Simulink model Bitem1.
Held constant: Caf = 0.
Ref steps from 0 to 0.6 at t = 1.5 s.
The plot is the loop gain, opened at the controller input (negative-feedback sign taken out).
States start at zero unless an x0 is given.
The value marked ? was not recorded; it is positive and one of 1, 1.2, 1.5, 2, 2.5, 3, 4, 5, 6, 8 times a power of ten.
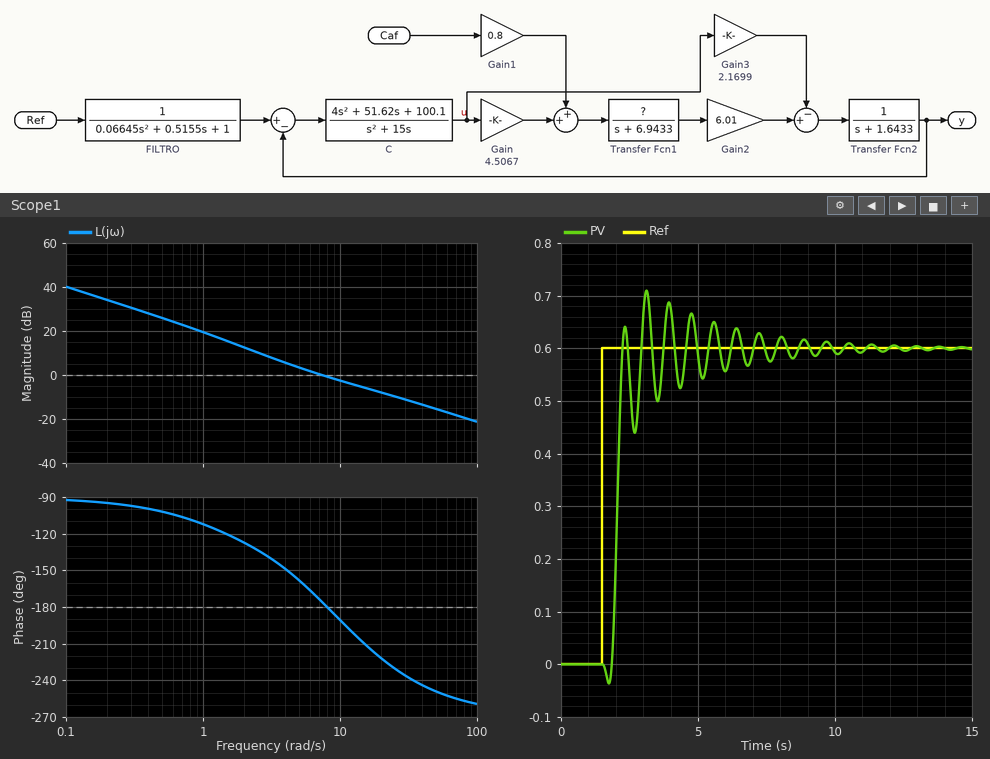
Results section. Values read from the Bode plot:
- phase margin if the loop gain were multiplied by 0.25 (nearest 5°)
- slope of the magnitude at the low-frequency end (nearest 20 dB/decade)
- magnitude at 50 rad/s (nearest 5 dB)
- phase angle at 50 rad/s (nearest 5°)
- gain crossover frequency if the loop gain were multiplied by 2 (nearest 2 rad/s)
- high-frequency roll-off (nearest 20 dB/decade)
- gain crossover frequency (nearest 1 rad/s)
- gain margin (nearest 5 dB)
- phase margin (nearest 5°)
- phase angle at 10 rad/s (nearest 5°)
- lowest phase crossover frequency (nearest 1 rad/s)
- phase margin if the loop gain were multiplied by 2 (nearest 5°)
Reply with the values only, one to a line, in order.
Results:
50°
-20 dB/decade
-15 dB
-250°
16 rad/s
-20 dB/decade
7 rad/s
0 dB
5°
-190°
8 rad/s
-30°
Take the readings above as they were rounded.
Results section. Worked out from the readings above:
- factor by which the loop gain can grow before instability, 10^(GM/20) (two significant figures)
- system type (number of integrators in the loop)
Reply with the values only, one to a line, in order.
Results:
1.0
1
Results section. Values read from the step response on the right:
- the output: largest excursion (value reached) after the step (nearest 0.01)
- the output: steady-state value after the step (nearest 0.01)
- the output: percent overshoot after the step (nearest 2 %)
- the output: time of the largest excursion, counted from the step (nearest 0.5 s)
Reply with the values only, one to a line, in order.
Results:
0.71
0.60
18 %
1.5 s
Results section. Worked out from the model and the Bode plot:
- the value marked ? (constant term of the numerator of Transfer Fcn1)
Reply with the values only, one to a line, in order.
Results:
1.2
